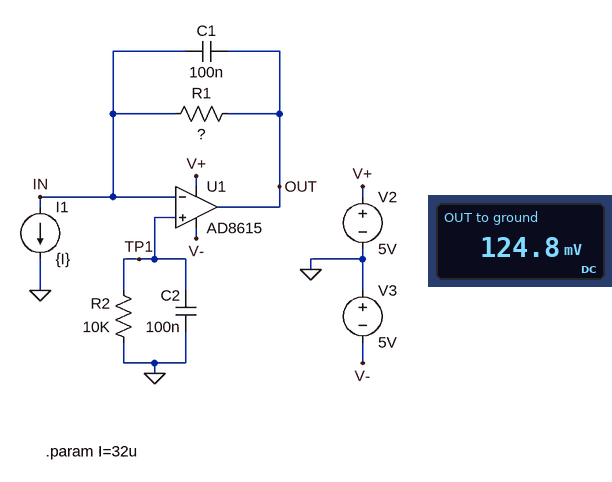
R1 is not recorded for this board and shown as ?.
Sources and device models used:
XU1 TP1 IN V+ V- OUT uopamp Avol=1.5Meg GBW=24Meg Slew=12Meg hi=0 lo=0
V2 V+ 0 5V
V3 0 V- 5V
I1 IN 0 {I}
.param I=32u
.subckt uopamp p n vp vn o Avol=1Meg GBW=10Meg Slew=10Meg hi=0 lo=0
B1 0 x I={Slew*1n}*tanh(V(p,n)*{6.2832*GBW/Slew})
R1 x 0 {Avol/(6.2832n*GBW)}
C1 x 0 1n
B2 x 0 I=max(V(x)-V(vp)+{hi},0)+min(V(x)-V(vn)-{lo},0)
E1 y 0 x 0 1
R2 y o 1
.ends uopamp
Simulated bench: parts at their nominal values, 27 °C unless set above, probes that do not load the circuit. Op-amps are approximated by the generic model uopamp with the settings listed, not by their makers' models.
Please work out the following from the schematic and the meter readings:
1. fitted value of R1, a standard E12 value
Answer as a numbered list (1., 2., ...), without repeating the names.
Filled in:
1. 3.9 kΩ
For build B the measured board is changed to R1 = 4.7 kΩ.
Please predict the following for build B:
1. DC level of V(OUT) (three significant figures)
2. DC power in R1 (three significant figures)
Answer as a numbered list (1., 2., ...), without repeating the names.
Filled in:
1. 150 mV
2. 4.81 µW
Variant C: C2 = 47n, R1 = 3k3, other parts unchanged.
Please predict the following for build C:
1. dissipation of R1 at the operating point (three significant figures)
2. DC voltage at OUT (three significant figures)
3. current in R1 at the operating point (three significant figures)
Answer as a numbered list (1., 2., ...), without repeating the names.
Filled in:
1. 3.38 µW
2. 106 mV
3. 32.0 µA
